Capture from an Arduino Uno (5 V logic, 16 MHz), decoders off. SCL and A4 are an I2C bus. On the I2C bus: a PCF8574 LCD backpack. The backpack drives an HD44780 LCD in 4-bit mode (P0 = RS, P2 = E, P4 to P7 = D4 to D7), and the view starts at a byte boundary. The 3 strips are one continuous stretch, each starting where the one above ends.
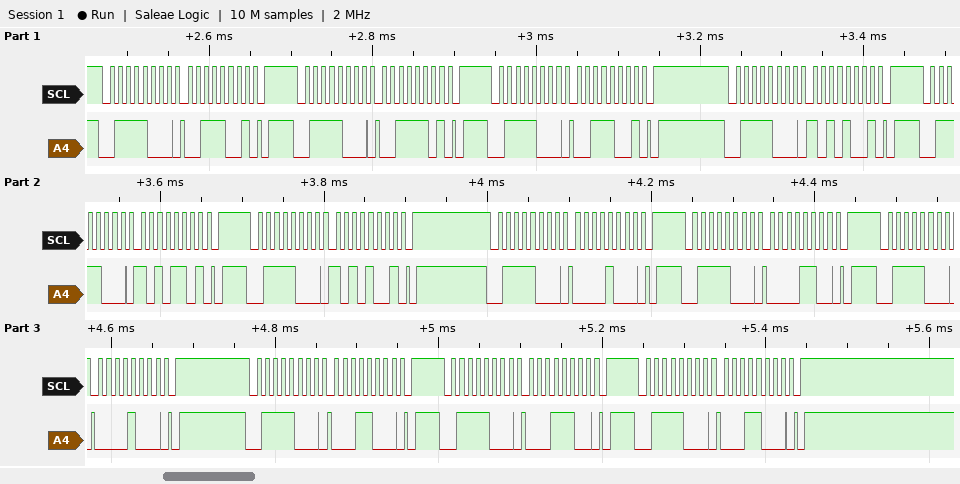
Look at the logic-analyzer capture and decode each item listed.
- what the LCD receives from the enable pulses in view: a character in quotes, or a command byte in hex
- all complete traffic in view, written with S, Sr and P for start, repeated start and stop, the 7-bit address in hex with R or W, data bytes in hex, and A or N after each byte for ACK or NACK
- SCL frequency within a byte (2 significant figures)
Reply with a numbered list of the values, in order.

1. ':' 0x01
2. S 3CW A 39 A P S 3CW A 3D A P S 3CW A 39 A P S 3CW A A9 A P S 3CW A AD A P S 3CW A A9 A P S 3CW A 08 A P S 3CW A 0C A P S 3CW A 08 A P S 3CW A 18 A P S 3CW A 1C A P S 3CW A 18 A P
3. 100 kHz
